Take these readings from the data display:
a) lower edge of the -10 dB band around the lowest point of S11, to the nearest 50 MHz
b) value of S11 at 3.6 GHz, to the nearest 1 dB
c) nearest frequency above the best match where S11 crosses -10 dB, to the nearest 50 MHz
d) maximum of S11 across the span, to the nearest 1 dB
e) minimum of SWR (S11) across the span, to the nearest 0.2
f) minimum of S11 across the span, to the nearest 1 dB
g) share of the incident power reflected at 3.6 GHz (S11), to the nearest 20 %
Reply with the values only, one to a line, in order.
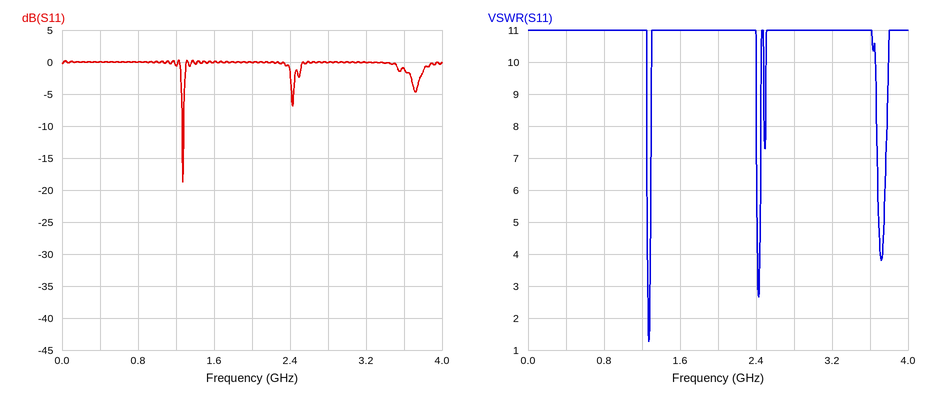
1.25 GHz
-1 dB
1.30 GHz
0 dB
1.2
-19 dB
80 %
